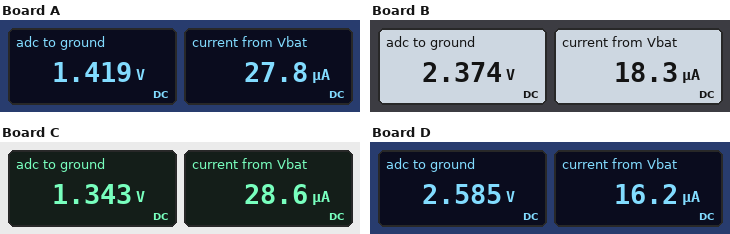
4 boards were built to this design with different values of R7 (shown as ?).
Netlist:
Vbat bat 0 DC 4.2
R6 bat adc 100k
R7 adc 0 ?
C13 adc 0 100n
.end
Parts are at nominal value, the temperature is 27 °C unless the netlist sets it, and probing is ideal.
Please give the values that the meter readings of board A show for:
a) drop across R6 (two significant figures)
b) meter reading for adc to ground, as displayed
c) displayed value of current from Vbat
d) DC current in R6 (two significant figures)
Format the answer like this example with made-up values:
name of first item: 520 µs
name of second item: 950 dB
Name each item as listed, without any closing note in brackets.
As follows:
drop across R6: 2.8 V
meter reading for adc to ground, as displayed: 1.419 V
displayed value of current from Vbat: 27.8 µA
DC current in R6: 28 µA
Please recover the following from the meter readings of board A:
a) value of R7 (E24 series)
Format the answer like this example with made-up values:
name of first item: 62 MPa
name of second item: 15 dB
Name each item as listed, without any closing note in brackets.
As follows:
value of R7: 51 kΩ
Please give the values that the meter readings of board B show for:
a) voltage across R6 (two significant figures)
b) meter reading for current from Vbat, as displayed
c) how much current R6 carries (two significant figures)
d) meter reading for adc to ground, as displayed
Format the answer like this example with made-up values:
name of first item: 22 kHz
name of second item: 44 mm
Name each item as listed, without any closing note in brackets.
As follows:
voltage across R6: 1.8 V
meter reading for current from Vbat, as displayed: 18.3 µA
how much current R6 carries: 18 µA
meter reading for adc to ground, as displayed: 2.374 V
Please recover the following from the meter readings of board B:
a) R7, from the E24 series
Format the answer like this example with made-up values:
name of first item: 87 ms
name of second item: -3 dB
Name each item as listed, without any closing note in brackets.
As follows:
R7, from the E24 series: 130 kΩ
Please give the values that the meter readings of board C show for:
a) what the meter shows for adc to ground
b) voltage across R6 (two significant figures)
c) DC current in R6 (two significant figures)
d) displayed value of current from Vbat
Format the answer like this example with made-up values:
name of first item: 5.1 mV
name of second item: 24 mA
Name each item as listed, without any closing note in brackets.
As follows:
what the meter shows for adc to ground: 1.343 V
voltage across R6: 2.9 V
DC current in R6: 29 µA
displayed value of current from Vbat: 28.6 µA
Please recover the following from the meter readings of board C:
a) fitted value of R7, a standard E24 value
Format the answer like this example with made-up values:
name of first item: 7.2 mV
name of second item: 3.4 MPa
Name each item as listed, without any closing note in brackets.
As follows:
fitted value of R7, a standard E24 value: 47 kΩ
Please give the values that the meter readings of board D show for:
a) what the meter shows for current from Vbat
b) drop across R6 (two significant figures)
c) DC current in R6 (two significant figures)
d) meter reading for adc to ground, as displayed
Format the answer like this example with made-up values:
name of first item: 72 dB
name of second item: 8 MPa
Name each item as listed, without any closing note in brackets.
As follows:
what the meter shows for current from Vbat: 16.2 µA
drop across R6: 1.6 V
DC current in R6: 16 µA
meter reading for adc to ground, as displayed: 2.585 V
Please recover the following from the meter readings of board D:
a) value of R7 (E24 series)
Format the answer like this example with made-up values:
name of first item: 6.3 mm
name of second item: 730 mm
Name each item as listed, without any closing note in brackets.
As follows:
value of R7: 160 kΩ
